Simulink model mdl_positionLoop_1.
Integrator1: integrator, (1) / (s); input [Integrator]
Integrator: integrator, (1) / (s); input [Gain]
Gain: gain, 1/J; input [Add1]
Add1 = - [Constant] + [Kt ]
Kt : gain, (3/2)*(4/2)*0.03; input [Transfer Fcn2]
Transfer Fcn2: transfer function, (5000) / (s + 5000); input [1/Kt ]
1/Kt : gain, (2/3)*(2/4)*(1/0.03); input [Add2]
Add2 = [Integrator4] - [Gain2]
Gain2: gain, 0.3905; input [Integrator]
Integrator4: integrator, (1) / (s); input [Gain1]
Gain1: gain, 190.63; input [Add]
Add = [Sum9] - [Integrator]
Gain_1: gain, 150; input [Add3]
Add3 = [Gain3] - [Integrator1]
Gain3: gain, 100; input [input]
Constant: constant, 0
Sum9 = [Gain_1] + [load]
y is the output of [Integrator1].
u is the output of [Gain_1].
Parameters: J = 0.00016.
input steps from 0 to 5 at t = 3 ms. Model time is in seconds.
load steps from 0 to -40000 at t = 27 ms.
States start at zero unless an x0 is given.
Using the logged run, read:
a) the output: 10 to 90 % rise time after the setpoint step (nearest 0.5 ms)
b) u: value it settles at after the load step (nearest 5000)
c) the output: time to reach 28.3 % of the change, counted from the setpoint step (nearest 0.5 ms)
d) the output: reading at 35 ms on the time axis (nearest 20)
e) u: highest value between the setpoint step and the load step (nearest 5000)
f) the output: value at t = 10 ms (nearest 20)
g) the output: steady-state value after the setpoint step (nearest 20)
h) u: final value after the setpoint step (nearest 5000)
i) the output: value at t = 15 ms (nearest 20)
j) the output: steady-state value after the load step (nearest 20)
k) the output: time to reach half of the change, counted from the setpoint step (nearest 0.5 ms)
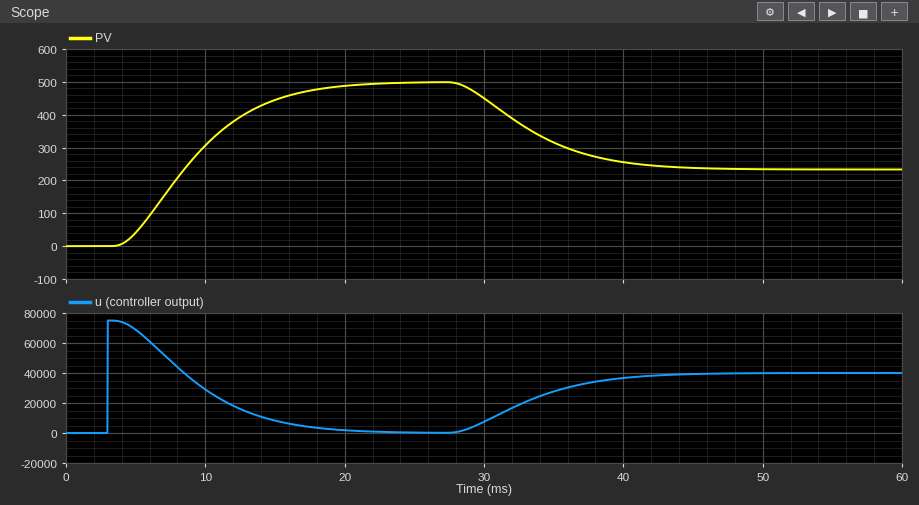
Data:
10.0 ms
40000
4.0 ms
320
75000
300
500
0
440
240
6.0 ms
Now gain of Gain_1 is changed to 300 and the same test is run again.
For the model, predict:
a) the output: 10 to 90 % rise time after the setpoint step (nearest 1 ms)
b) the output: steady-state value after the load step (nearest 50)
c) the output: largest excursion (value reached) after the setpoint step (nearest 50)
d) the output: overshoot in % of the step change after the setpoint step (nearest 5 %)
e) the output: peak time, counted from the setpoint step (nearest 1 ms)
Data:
4 ms
350
550
10 %
10 ms
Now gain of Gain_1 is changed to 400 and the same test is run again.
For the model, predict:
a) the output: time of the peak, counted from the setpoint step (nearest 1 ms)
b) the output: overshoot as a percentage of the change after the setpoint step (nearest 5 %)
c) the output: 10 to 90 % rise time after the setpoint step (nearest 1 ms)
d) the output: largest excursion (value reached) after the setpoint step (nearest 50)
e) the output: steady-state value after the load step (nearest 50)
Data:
8 ms
15 %
3 ms
600
400
